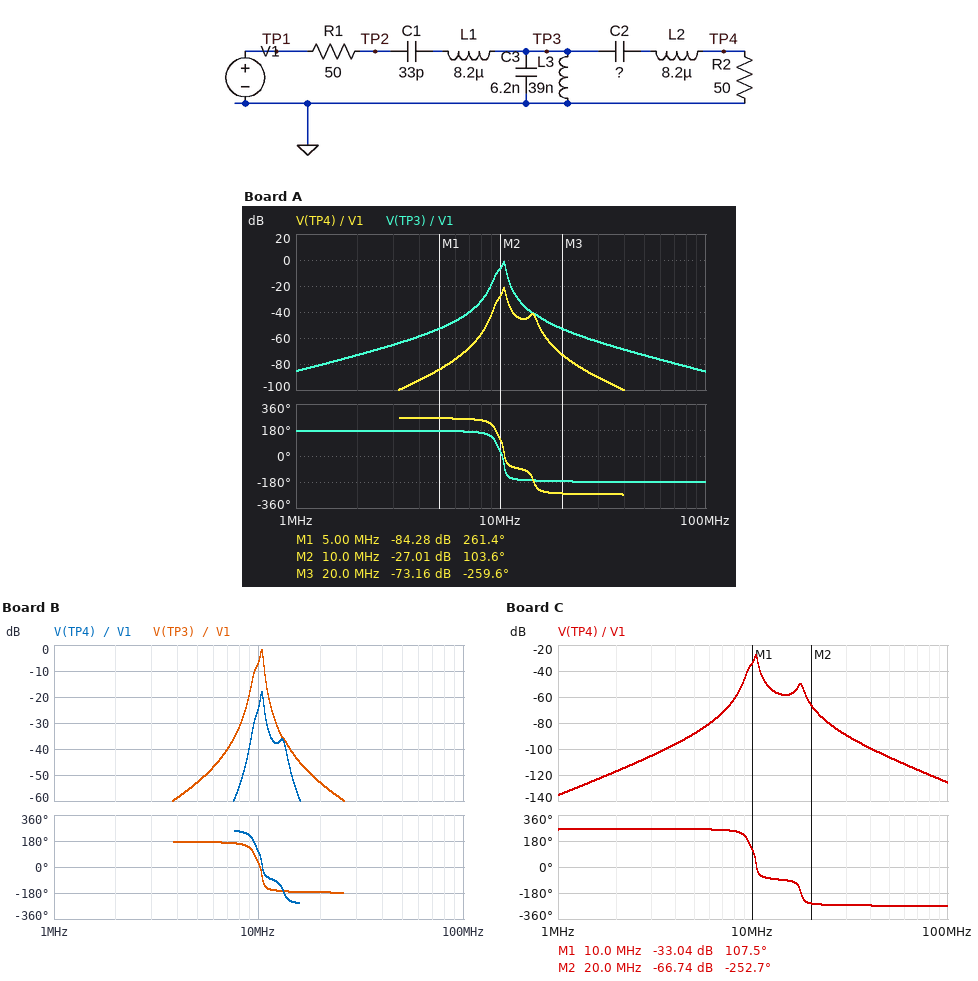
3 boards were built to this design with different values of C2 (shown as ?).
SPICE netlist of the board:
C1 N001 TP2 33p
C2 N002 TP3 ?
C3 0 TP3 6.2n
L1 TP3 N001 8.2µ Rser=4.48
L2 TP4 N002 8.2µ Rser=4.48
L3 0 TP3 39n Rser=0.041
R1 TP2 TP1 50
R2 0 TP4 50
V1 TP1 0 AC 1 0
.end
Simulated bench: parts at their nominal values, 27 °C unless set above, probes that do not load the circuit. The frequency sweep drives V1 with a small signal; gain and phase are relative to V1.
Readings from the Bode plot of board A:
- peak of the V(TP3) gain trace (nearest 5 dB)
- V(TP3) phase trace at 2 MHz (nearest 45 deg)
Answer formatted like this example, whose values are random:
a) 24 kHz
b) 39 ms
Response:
a) 0 dB
b) 180 deg
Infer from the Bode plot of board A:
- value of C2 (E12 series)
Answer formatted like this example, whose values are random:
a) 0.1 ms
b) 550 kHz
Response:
a) 15 pF
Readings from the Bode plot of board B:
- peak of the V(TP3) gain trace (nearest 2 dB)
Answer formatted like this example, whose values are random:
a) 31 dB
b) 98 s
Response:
a) -2 dB
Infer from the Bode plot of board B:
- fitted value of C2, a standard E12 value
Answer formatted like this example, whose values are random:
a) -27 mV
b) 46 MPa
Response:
a) 18 pF
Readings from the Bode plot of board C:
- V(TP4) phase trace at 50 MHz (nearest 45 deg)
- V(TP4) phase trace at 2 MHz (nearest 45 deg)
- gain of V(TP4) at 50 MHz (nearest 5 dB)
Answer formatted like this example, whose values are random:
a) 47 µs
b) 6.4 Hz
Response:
a) -270 deg
b) 270 deg
c) -105 dB
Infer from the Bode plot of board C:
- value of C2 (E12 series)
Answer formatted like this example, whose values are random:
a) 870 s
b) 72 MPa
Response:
a) 10 pF
